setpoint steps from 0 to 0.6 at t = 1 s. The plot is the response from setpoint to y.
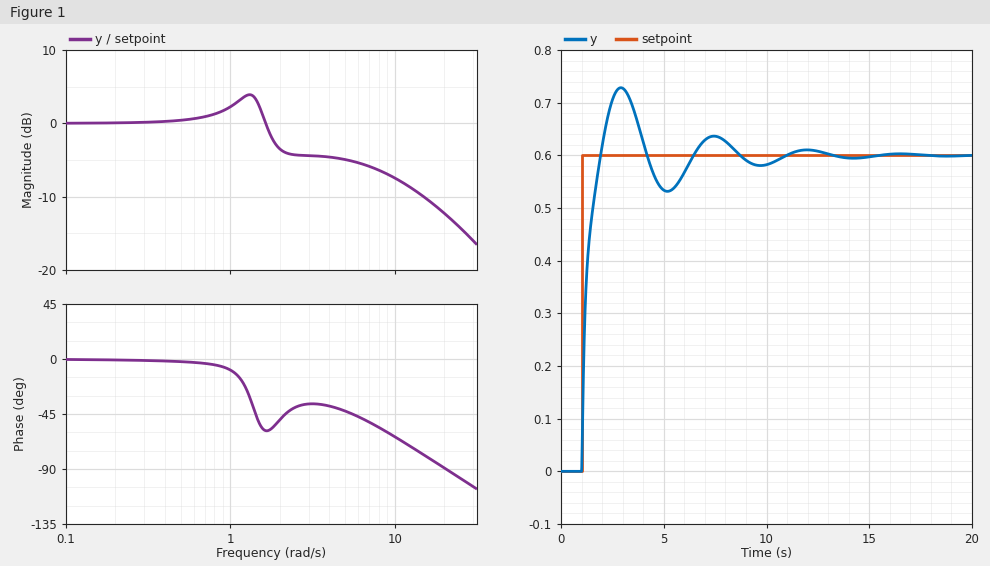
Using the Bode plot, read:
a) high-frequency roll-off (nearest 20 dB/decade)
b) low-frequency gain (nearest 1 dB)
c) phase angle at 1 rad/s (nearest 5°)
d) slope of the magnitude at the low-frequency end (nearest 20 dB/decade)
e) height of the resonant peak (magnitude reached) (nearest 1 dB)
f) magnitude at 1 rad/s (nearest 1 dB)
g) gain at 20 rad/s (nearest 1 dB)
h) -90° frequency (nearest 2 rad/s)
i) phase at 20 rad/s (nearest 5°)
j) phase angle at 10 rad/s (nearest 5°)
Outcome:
-20 dB/decade
0 dB
-10°
0 dB/decade
4 dB
2 dB
-12 dB
20 rad/s
-90°
-65°
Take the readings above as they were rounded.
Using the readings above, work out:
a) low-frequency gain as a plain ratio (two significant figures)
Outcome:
1.0
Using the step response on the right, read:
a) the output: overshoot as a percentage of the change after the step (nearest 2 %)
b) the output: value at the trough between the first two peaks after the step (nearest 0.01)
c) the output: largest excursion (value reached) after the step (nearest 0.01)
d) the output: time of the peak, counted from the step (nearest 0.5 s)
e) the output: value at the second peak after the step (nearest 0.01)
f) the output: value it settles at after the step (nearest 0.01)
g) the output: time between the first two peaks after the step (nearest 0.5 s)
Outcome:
22 %
0.53
0.73
2.0 s
0.64
0.60
4.5 s
